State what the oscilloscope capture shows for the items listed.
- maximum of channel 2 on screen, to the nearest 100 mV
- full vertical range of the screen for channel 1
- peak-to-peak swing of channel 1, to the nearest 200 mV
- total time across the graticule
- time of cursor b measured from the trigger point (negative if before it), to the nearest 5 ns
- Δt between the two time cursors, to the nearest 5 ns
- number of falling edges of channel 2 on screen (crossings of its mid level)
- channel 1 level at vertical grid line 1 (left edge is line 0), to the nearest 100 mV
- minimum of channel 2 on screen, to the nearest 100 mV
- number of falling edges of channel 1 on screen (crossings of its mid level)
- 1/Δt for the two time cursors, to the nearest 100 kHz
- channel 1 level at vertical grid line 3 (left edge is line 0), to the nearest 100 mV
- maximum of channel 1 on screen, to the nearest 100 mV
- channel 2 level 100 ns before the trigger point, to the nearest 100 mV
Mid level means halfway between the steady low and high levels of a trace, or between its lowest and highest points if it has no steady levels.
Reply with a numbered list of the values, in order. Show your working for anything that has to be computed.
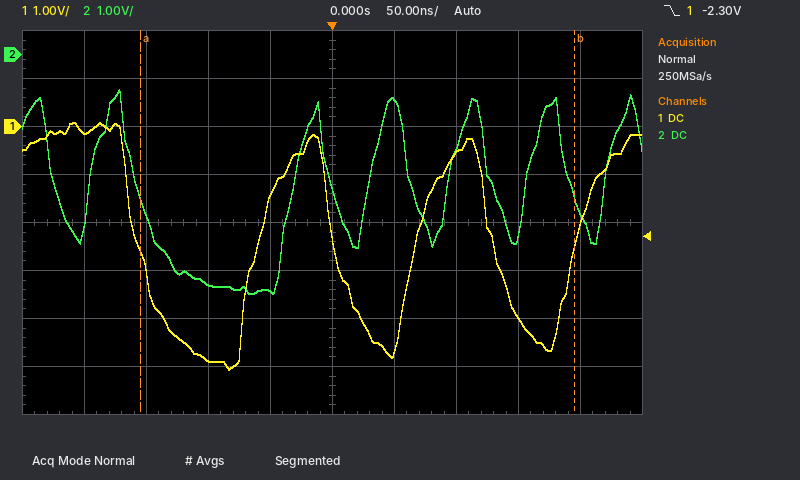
1. -700 mV
2. 8 V
3. 5.2 V
4. 500 ns
5. +195 ns
6. 350 ns
7. 6
8. -100 mV
9. -5.0 V
10. 3
11. 1 / 350 ns ≈ 2.9 MHz
12. -4.9 V
13. 100 mV
14. -4.8 V
